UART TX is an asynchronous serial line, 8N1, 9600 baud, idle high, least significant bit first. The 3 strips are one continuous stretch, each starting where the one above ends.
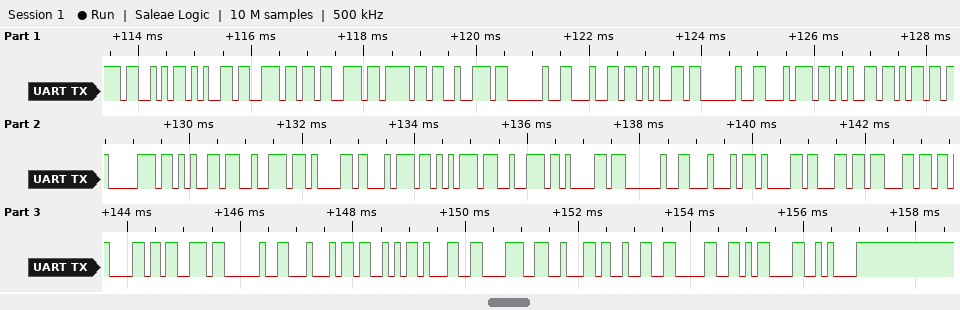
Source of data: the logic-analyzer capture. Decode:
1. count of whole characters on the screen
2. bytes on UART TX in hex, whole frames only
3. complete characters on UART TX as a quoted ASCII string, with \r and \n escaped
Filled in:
38
53 65 6E 73 6F 72 20 64 65 20 74 65 6D 70 65 72 61 74 75 72 61 20 44 61 6C 6C 61 73 20 44 53 31 38 62 32 30 0D 0A
"Sensor de temperatura Dallas DS18b20\r\n"
